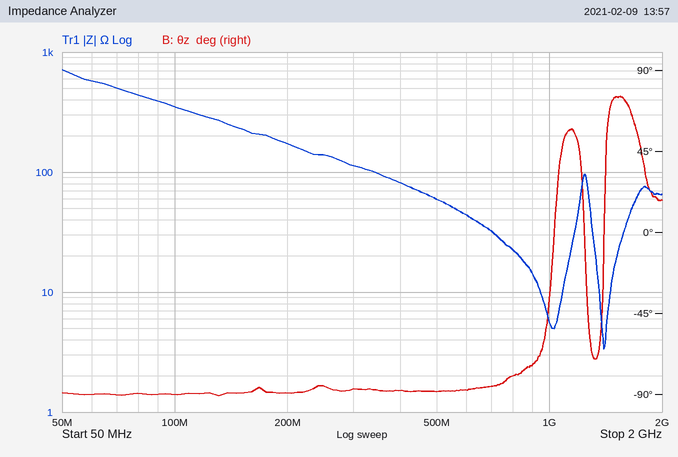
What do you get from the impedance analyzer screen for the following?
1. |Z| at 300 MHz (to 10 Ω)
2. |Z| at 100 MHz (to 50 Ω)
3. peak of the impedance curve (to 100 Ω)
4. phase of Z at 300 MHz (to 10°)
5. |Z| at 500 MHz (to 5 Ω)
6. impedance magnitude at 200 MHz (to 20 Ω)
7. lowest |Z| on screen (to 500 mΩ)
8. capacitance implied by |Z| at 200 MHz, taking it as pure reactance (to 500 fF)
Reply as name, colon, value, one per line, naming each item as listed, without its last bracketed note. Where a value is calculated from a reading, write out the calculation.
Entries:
|Z| at 300 MHz: 110 Ω
|Z| at 100 MHz: 350 Ω
peak of the impedance curve: 700 Ω
phase of Z at 300 MHz: -90°
|Z| at 500 MHz: 60 Ω
impedance magnitude at 200 MHz: 180 Ω
lowest |Z| on screen: 3.5 Ω
capacitance implied by |Z| at 200 MHz, taking it as pure reactance: C = 1/(2π × 200 MHz × 180 Ω) ≈ 4.42 pF, so 4.5 pF to the nearest 500 fF
